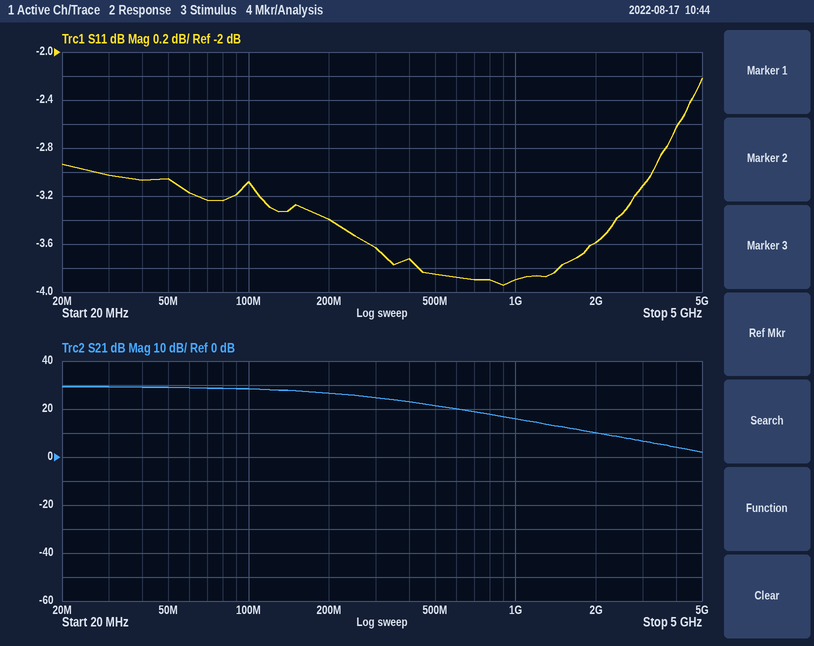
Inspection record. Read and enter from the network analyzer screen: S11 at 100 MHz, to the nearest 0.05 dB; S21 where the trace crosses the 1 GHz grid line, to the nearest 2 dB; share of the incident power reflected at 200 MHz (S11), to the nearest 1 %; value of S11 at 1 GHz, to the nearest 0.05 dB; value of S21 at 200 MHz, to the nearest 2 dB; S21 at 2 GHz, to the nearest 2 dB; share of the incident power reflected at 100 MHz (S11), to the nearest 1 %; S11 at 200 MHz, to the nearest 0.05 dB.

-3.10 dB
16 dB
46 %
-3.90 dB
26 dB
10 dB
49 %
-3.40 dB
